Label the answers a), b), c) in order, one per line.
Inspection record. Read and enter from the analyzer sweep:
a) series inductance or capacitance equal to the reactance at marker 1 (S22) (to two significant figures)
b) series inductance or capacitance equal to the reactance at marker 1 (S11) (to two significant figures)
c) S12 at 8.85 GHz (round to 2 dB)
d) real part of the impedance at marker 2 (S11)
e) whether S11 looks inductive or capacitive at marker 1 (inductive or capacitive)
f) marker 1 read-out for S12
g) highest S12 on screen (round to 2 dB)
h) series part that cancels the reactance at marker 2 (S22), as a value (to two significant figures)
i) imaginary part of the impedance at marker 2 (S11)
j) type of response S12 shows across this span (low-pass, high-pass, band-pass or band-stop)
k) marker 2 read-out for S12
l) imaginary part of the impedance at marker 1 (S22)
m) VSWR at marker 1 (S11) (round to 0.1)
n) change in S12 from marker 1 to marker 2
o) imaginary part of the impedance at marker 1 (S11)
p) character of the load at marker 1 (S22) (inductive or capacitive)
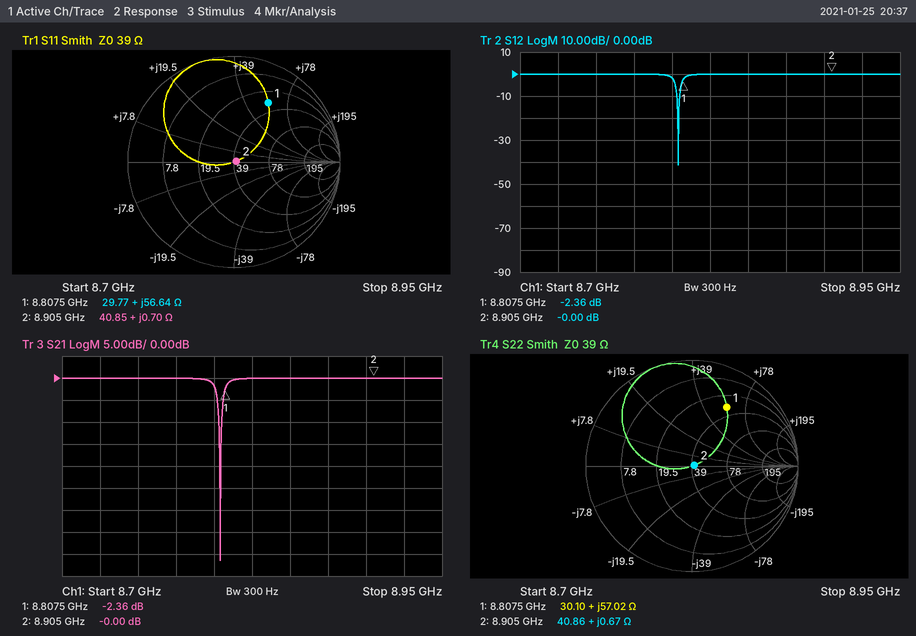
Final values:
a) 1.0 nH
b) 1.0 nH
c) 0 dB
d) 40.85 Ω
e) inductive
f) -2.36 dB
g) 0 dB
h) 27 pF
i) +0.70 Ω
j) band-stop
k) -0.00 dB
l) +57.02 Ω
m) 4.6
n) 2.36 dB
o) +56.64 Ω
p) inductive
